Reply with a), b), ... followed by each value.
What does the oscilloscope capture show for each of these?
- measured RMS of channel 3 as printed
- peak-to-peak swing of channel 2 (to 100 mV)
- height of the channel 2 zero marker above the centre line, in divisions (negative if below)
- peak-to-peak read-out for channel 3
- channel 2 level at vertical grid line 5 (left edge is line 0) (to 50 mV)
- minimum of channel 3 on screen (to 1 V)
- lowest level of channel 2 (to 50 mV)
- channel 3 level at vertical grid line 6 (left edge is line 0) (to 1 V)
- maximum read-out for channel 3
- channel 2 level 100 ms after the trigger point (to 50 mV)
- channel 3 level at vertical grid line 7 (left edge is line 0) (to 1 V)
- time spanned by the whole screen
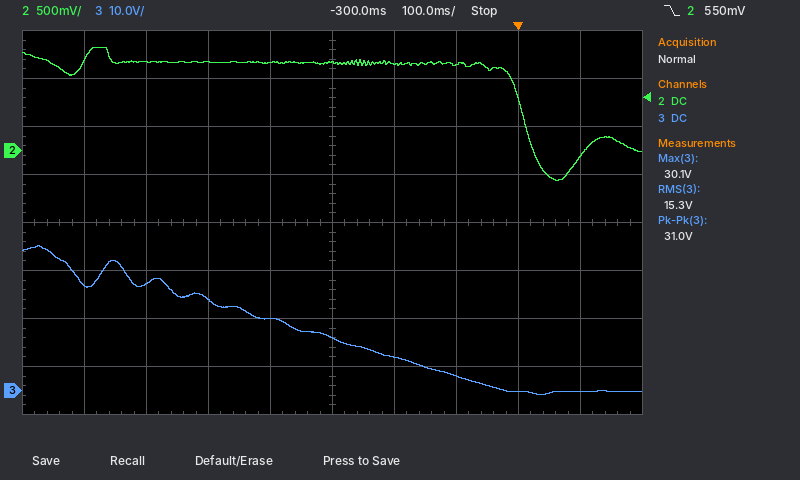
a) 15.3 V
b) 1.40 V
c) +1.5 div
d) 31.0 V
e) 900 mV
f) -1 V
g) -300 mV
h) 7 V
i) 30.1 V
j) -50 mV
k) 3 V
l) 1 s
